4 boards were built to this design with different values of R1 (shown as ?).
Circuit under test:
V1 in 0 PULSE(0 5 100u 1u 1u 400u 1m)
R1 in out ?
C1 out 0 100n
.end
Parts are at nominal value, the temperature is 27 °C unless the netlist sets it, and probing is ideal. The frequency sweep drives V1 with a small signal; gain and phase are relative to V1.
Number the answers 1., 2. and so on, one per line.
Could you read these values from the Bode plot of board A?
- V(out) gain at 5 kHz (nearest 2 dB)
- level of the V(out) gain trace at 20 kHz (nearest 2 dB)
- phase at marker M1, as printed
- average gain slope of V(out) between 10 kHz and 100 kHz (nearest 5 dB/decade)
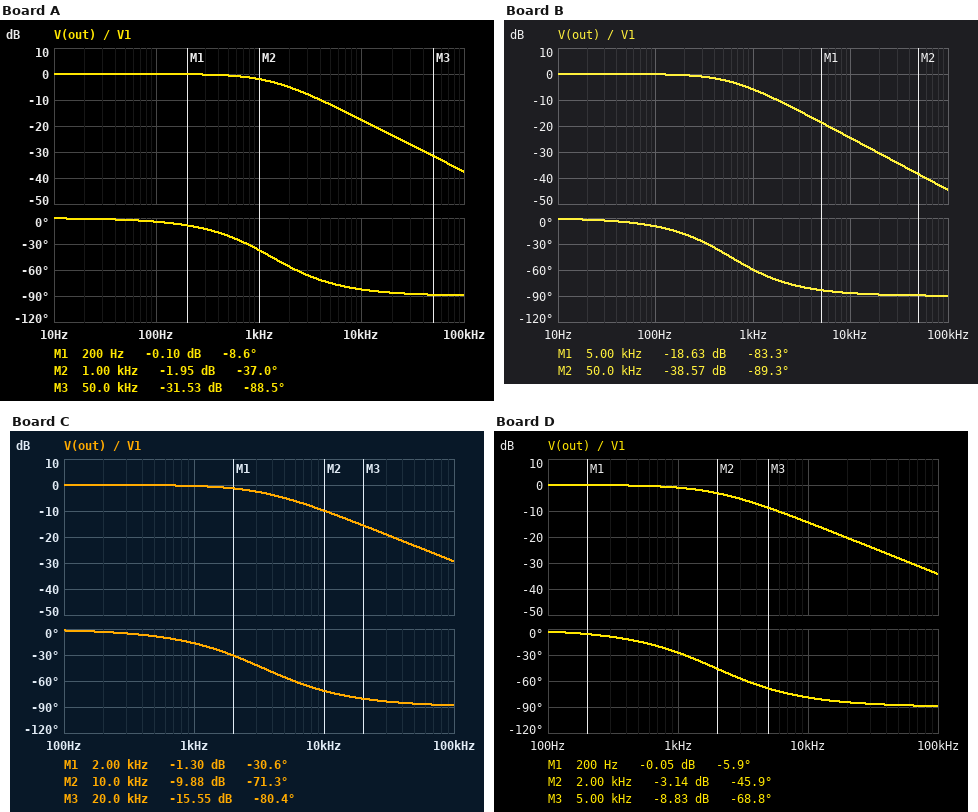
1. -12 dB
2. -24 dB
3. -8.6 deg
4. -20 dB/decade
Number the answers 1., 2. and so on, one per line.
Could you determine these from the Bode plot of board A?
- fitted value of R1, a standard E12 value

1. 1.2 kΩ
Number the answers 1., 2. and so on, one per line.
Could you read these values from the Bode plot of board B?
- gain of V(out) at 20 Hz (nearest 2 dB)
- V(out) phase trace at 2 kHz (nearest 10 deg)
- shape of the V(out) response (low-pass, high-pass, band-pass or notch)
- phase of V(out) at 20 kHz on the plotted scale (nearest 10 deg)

1. 0 dB
2. -70 deg
3. low-pass
4. -90 deg
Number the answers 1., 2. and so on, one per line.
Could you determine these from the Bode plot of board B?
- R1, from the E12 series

1. 2.7 kΩ
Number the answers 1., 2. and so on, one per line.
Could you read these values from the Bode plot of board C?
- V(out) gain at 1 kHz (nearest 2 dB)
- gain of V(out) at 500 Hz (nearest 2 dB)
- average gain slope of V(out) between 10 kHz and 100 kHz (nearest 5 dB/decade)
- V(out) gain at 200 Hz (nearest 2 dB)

1. 0 dB
2. 0 dB
3. -20 dB/decade
4. 0 dB
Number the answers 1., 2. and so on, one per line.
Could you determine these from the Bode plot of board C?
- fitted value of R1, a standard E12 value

1. 470 Ω
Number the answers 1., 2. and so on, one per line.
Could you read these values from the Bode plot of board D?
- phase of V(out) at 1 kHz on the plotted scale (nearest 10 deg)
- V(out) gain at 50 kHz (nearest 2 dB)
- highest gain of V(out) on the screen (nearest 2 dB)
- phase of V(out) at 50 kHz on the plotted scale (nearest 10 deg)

1. -30 deg
2. -28 dB
3. 0 dB
4. -90 deg
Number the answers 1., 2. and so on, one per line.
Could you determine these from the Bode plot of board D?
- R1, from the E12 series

1. 820 Ω
